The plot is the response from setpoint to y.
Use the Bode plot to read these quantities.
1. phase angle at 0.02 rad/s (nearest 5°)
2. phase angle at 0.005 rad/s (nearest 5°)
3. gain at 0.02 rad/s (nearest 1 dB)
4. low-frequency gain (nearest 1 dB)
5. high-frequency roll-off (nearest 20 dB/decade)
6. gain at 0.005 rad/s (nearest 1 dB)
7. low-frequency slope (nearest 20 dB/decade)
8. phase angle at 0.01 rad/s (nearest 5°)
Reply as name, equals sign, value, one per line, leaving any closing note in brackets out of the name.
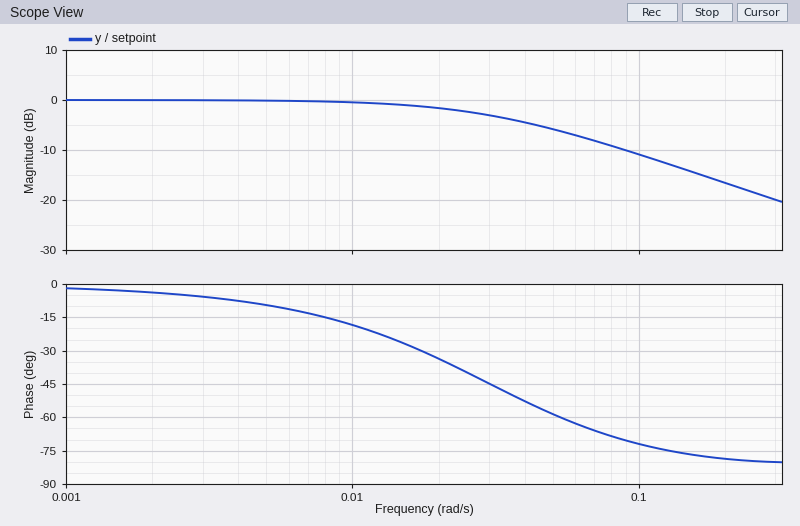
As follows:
phase angle at 0.02 rad/s = -35°
phase angle at 0.005 rad/s = -10°
gain at 0.02 rad/s = -2 dB
low-frequency gain = 0 dB
high-frequency roll-off = -20 dB/decade
gain at 0.005 rad/s = 0 dB
low-frequency slope = 0 dB/decade
phase angle at 0.01 rad/s = -20°
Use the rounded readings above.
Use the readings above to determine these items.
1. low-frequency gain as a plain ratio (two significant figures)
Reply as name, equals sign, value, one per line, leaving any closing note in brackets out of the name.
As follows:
low-frequency gain as a plain ratio = 1.0
